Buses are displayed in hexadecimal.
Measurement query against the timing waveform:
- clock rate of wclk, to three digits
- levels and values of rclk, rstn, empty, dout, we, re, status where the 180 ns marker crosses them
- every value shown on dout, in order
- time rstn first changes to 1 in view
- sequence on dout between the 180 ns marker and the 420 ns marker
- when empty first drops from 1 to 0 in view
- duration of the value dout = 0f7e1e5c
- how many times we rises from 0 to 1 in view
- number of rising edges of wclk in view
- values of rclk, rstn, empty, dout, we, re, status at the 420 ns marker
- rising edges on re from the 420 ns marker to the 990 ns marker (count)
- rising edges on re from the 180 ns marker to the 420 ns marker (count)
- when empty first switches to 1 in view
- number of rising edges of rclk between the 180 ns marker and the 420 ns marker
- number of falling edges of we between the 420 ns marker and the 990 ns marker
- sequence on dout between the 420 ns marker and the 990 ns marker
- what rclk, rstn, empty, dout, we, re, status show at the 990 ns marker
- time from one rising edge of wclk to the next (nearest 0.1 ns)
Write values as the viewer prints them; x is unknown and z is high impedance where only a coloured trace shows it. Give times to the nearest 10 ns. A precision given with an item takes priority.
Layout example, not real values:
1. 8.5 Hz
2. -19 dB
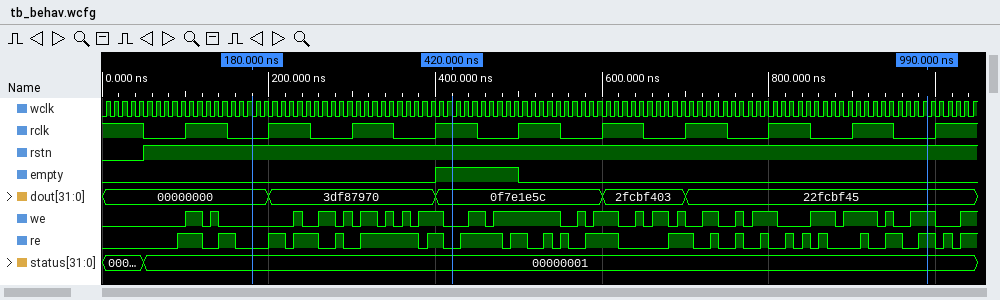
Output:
1. 100 MHz
2. rclk=0, rstn=1, empty=0, dout=00000000, we=0, re=0, status=00000001
3. 00000000, 3df87970, 0f7e1e5c, 2fcbf403, 22fcbf45
4. 50 ns
5. 00000000, 3df87970, 0f7e1e5c
6. 500 ns
7. 200 ns
8. 24
9. 105
10. rclk=1, rstn=1, empty=1, dout=0f7e1e5c, we=0, re=0, status=00000001
11. 15
12. 5
13. 400 ns
14. 3
15. 13
16. 0f7e1e5c, 2fcbf403, 22fcbf45
17. rclk=0, rstn=1, empty=0, dout=22fcbf45, we=1, re=1, status=00000001
18. 10 ns
